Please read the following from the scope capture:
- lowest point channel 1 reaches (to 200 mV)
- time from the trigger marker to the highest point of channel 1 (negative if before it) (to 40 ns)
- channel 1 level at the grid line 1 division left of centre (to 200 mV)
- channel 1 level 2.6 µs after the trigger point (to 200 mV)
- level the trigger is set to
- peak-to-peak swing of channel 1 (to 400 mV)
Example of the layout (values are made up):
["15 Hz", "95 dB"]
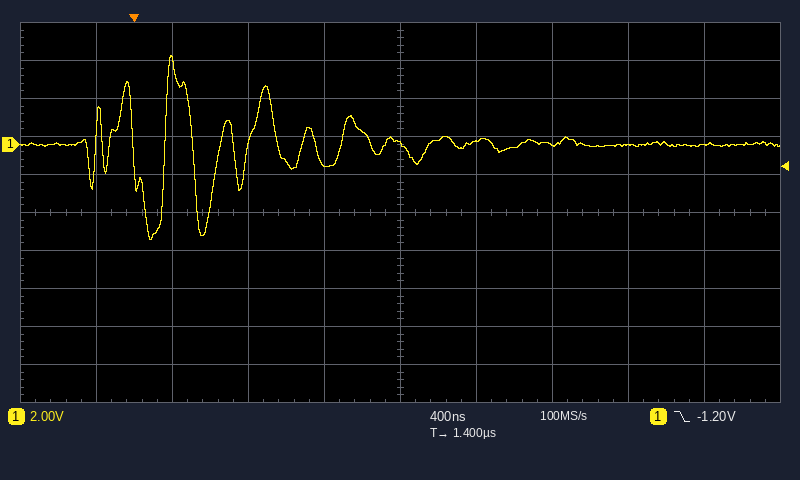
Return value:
["-5.0 V", "+200 ns", "-1.0 V", "0.0 V", "-1.20 V", "9.6 V"]
